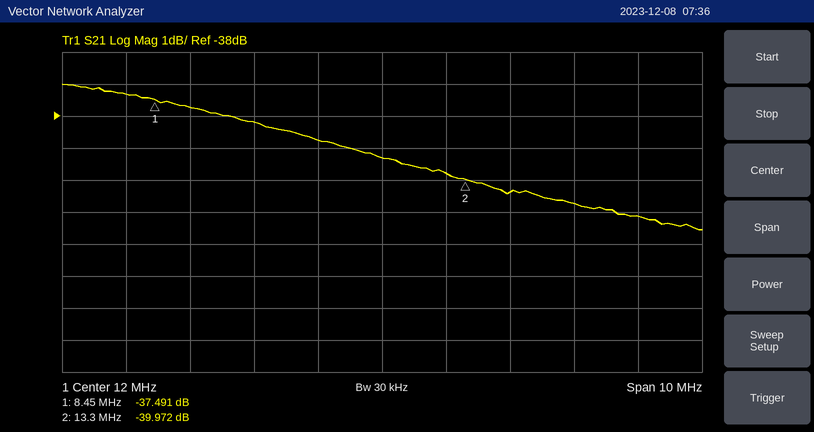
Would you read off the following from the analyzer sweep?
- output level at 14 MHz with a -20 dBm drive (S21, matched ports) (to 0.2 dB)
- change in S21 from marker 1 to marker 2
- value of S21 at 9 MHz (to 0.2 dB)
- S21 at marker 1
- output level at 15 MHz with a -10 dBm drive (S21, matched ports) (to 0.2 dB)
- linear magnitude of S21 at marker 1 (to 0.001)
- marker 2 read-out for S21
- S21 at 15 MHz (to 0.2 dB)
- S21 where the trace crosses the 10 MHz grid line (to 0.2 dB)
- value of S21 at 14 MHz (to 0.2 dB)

-60.4 dBm
-2.481 dB
-37.8 dB
-37.491 dB
-50.8 dBm
0.013
-39.972 dB
-40.8 dB
-38.2 dB
-40.4 dB
